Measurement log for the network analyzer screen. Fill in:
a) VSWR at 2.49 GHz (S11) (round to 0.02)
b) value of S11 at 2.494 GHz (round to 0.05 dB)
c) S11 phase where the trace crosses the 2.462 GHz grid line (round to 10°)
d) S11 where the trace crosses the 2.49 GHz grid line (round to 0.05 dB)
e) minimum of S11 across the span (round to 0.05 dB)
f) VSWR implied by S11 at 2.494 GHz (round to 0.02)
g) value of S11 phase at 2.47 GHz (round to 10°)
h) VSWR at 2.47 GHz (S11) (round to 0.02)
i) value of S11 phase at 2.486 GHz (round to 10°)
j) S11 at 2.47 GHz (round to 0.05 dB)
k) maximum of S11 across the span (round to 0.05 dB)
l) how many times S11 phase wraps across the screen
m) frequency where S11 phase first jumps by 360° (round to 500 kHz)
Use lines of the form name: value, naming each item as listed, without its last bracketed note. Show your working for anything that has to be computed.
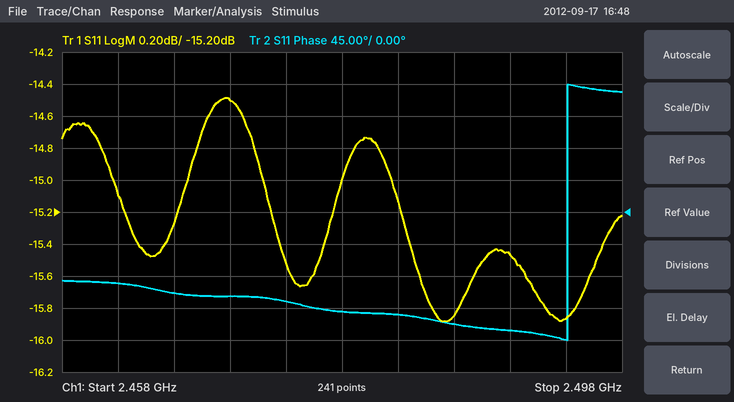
VSWR at 2.49 GHz (S11): |Γ| = 10^(-15.45/20) = 0.1688; VSWR = (1 + 0.1688)/(1 − 0.1688) ≈ 1.41, so 1.40 to the nearest 0.02
value of S11 at 2.494 GHz: -15.85 dB
S11 phase where the trace crosses the 2.462 GHz grid line: -100°
S11 where the trace crosses the 2.49 GHz grid line: -15.45 dB
minimum of S11 across the span: -15.90 dB
VSWR implied by S11 at 2.494 GHz: |Γ| = 10^(-15.85/20) = 0.1613; VSWR = (1 + 0.1613)/(1 − 0.1613) ≈ 1.38
value of S11 phase at 2.47 GHz: -120°
VSWR at 2.47 GHz (S11): |Γ| = 10^(-14.5/20) = 0.1884; VSWR = (1 + 0.1884)/(1 − 0.1884) ≈ 1.46
value of S11 phase at 2.486 GHz: -160°
S11 at 2.47 GHz: -14.50 dB
maximum of S11 across the span: -14.50 dB
how many times S11 phase wraps across the screen: 1
frequency where S11 phase first jumps by 360°: 2.4940 GHz
